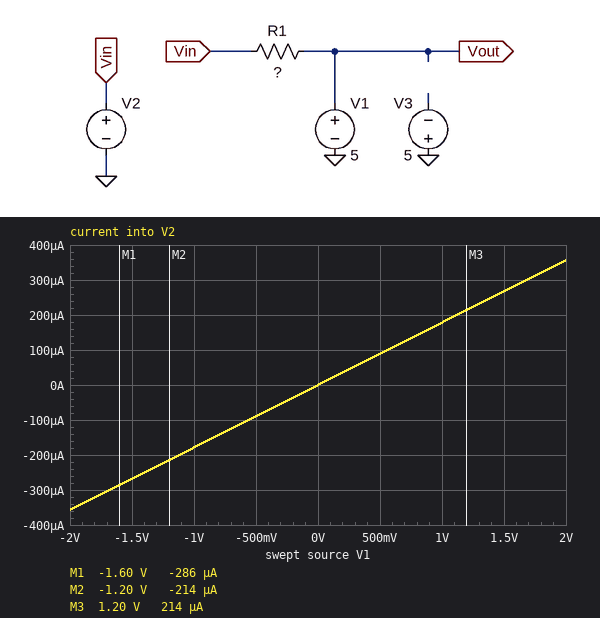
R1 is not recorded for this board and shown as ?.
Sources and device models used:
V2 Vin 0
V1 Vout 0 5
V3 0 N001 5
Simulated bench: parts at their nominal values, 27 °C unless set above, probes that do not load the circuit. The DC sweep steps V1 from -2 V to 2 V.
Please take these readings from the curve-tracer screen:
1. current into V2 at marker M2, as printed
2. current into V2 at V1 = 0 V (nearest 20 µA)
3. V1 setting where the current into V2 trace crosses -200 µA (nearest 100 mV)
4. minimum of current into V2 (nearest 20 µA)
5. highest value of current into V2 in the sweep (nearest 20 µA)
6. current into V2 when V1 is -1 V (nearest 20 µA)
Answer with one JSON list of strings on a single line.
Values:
["-214 µA", "0 A", "-1.1 V", "-360 µA", "360 µA", "-180 µA"]
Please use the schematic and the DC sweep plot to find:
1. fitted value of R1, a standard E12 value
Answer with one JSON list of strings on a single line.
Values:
["5.6 kΩ"]
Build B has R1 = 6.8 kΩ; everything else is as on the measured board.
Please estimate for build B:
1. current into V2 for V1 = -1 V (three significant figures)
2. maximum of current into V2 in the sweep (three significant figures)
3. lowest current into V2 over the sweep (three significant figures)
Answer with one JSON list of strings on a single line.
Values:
["-147 µA", "294 µA", "-294 µA"]
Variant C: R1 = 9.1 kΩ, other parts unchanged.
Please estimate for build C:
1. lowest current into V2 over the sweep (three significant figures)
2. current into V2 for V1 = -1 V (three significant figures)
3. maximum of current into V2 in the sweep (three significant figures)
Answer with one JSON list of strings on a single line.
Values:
["-220 µA", "-110 µA", "220 µA"]
